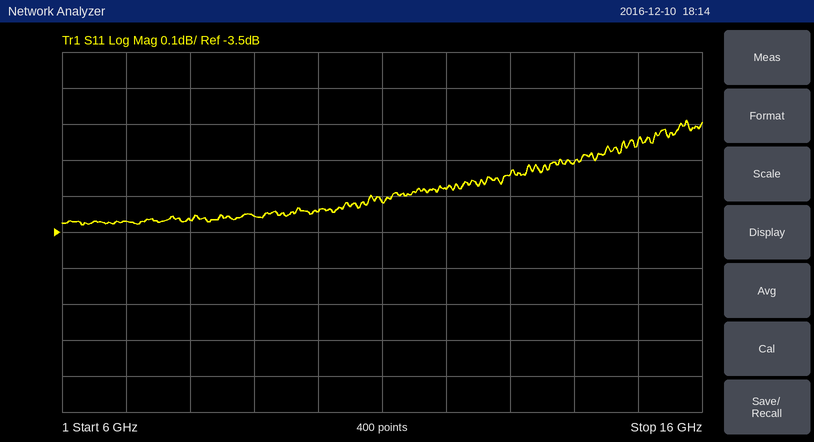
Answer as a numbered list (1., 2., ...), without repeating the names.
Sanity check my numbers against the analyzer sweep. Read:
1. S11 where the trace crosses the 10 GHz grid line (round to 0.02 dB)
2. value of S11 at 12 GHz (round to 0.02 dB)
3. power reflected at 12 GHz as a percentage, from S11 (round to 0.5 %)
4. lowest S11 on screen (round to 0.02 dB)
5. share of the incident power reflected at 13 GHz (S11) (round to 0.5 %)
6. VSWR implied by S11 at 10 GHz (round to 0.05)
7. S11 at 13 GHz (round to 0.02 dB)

1. -3.44 dB
2. -3.38 dB
3. 46.0 %
4. -3.48 dB
5. 46.5 %
6. 5.10
7. -3.34 dB
